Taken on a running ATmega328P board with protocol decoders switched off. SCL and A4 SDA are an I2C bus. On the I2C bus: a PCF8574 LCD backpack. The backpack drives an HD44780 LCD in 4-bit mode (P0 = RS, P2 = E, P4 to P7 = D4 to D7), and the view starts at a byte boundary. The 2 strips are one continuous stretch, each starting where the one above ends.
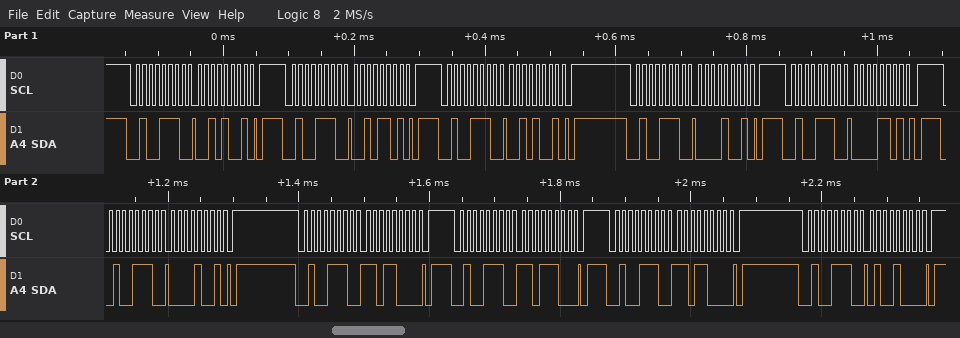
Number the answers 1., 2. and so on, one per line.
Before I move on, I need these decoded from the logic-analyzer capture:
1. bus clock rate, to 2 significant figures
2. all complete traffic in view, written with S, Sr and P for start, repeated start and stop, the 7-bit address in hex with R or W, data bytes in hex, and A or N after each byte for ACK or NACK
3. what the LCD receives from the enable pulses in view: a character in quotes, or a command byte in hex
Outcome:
1. 100 kHz
2. S 27W A 29 A P S 27W A 2D A P S 27W A 29 A P S 27W A 09 A P S 27W A 0D A P S 27W A 09 A P S 27W A D8 A P S 27W A DC A P S 27W A D8 A P S 27W A 48 A P
3. ' '
